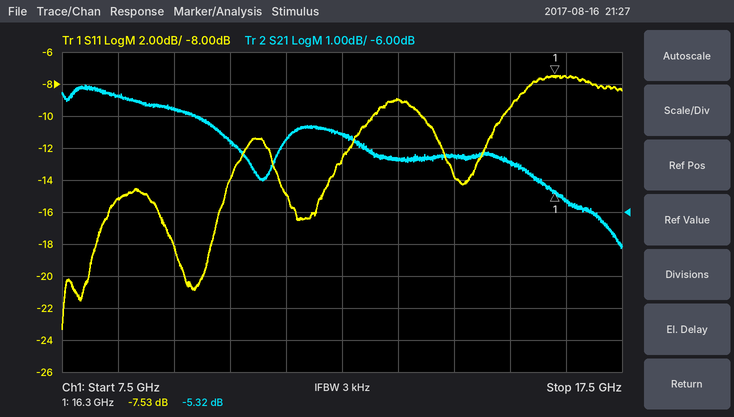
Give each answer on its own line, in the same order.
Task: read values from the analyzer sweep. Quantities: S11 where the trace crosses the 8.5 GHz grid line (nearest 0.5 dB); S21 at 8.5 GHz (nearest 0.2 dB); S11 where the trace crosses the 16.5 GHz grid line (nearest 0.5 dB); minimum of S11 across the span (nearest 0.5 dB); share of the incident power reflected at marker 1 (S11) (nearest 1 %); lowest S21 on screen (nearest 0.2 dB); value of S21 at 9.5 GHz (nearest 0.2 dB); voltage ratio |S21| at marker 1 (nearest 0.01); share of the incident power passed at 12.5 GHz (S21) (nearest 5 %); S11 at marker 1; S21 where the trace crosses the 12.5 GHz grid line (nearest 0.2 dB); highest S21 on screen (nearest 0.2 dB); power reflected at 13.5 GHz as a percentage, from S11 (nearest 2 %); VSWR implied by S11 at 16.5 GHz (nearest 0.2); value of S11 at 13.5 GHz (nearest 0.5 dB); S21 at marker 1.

-15.0 dB
-2.4 dB
-7.5 dB
-23.5 dB
18 %
-7.2 dB
-2.8 dB
0.54
45 %
-7.53 dB
-3.6 dB
-2.0 dB
12 %
2.4
-9.0 dB
-5.32 dB
